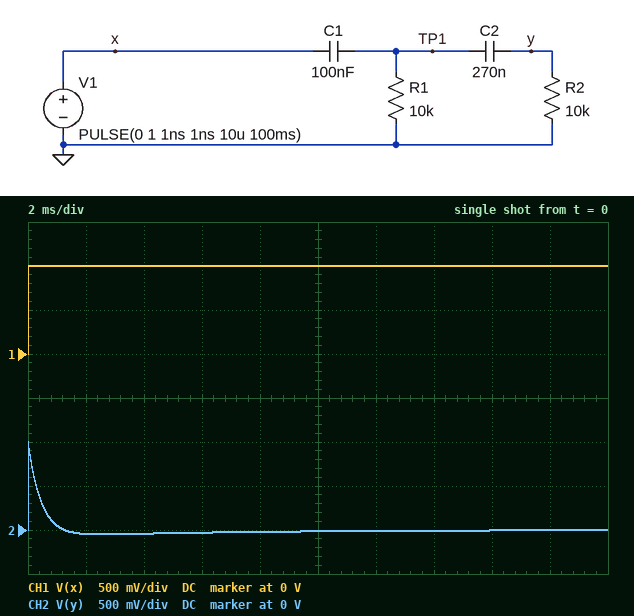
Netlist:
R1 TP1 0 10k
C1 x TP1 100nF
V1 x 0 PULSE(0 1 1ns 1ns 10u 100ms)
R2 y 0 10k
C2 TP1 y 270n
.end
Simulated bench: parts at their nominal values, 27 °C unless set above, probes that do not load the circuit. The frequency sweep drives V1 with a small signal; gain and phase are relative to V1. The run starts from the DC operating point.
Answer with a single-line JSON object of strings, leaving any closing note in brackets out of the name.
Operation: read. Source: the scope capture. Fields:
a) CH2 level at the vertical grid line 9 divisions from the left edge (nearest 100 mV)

{"CH2 level at the vertical grid line 9 divisions from the left edge": "0 V"}
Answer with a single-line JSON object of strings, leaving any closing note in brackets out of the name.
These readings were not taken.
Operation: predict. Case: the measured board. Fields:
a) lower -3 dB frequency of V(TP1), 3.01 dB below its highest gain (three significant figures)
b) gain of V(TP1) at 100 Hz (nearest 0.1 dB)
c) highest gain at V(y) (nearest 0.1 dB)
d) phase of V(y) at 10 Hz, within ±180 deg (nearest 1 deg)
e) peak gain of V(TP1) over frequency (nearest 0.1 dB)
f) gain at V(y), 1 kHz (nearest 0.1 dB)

{"lower -3 dB frequency of V(TP1), 3.01 dB below its highest gain": "343 Hz", "gain of V(TP1) at 100 Hz": "-10.2 dB", "highest gain at V(y)": "0 dB", "phase of V(y) at 10 Hz, within ±180 deg": "158 deg", "peak gain of V(TP1) over frequency": "0 dB", "gain at V(y), 1 kHz": "-0.5 dB"}
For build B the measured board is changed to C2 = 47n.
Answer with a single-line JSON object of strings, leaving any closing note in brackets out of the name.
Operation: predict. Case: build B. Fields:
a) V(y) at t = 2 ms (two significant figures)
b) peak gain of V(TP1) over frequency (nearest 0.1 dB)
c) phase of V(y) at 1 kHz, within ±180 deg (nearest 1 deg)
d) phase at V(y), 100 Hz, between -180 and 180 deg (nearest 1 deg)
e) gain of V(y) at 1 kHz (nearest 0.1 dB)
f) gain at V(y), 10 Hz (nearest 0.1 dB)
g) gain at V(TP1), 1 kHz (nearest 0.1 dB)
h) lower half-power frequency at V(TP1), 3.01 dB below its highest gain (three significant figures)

{"V(y) at t = 2 ms": "-61 mV", "peak gain of V(TP1) over frequency": "0 dB", "phase of V(y) at 1 kHz, within ±180 deg": "35 deg", "phase at V(y), 100 Hz, between -180 and 180 deg": "124 deg", "gain of V(y) at 1 kHz": "-1.2 dB", "gain at V(y), 10 Hz": "-54.7 dB", "gain at V(TP1), 1 kHz": "-0.8 dB", "lower half-power frequency at V(TP1), 3.01 dB below its highest gain": "345 Hz"}
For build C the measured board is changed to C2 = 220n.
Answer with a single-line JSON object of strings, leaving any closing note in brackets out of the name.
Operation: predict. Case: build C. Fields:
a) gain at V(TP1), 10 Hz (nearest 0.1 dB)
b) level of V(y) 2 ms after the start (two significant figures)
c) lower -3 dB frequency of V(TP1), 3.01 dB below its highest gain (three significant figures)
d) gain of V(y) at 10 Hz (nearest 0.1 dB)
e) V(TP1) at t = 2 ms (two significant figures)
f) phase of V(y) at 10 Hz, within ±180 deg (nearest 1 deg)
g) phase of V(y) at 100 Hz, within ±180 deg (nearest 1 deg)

{"gain at V(TP1), 10 Hz": "-24.4 dB", "level of V(y) 2 ms after the start": "-54 mV", "lower -3 dB frequency of V(TP1), 3.01 dB below its highest gain": "347 Hz", "gain of V(y) at 10 Hz": "-41.6 dB", "V(TP1) at t = 2 ms": "92 mV", "phase of V(y) at 10 Hz, within ±180 deg": "161 deg", "phase of V(y) at 100 Hz, within ±180 deg": "92 deg"}
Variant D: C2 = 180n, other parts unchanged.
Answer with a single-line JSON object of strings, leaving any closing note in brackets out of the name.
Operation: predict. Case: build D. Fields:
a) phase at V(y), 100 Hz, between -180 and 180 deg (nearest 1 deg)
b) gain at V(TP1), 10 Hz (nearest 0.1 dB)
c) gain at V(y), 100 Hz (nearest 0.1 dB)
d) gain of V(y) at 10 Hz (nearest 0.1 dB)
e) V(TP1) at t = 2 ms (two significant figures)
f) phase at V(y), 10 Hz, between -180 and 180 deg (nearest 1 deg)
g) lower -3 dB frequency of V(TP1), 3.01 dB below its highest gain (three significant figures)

{"phase at V(y), 100 Hz, between -180 and 180 deg": "96 deg", "gain at V(TP1), 10 Hz": "-24.3 dB", "gain at V(y), 100 Hz": "-12.2 dB", "gain of V(y) at 10 Hz": "-43.3 dB", "V(TP1) at t = 2 ms": "100 mV", "phase at V(y), 10 Hz, between -180 and 180 deg": "164 deg", "lower -3 dB frequency of V(TP1), 3.01 dB below its highest gain": "351 Hz"}
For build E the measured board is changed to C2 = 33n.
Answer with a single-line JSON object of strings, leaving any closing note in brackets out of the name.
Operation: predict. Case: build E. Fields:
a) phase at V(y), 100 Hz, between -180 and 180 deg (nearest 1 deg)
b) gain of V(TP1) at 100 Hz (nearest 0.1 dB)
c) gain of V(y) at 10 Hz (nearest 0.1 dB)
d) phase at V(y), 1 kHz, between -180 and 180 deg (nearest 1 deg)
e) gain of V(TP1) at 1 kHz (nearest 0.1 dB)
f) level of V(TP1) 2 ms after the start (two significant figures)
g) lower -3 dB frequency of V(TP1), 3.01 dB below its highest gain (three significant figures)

{"phase at V(y), 100 Hz, between -180 and 180 deg": "130 deg", "gain of V(TP1) at 100 Hz": "-6.5 dB", "gain of V(y) at 10 Hz": "-57.7 dB", "phase at V(y), 1 kHz, between -180 and 180 deg": "41 deg", "gain of V(TP1) at 1 kHz": "-0.8 dB", "level of V(TP1) 2 ms after the start": "160 mV", "lower -3 dB frequency of V(TP1), 3.01 dB below its highest gain": "298 Hz"}
